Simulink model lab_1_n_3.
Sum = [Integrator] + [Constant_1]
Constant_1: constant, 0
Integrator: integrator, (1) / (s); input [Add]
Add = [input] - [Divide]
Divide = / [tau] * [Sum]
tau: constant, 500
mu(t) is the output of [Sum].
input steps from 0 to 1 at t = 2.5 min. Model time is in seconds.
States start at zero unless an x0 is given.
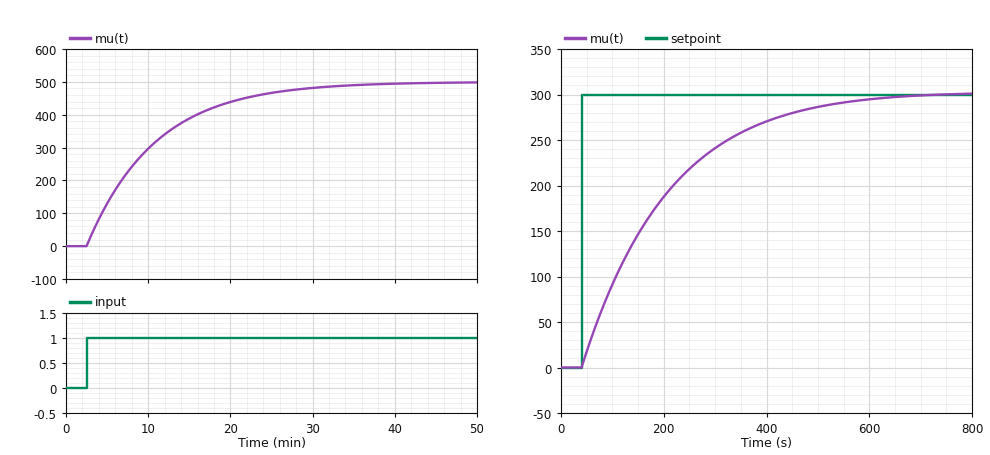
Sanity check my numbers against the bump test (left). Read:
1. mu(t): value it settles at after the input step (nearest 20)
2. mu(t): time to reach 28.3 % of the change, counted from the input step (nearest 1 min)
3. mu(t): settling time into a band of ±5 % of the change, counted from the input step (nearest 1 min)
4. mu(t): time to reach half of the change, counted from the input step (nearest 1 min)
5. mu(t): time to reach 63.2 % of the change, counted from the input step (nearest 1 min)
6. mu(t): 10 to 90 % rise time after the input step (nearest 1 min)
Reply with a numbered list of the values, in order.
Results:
1. 500
2. 3 min
3. 25 min
4. 6 min
5. 8 min
6. 18 min
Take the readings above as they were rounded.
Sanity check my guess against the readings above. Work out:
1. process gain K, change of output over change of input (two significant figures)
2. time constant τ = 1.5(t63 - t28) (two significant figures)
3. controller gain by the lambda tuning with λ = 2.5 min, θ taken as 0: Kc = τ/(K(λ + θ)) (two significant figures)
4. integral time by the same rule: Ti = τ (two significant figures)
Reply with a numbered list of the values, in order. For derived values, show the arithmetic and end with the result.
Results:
1. (500 - 0) / 1 = 500
2. 1.5 × (8 - 3) = 7.5 min
3. 7.5 / (500 × (2.5 + 0)) = 0.0060
4. 7.5 min
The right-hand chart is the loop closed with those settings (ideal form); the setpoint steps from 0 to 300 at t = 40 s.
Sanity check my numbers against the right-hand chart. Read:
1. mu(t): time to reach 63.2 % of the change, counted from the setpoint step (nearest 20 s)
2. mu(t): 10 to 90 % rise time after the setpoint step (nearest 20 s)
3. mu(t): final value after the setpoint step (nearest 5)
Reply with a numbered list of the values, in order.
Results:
1. 160 s
2. 340 s
3. 300
